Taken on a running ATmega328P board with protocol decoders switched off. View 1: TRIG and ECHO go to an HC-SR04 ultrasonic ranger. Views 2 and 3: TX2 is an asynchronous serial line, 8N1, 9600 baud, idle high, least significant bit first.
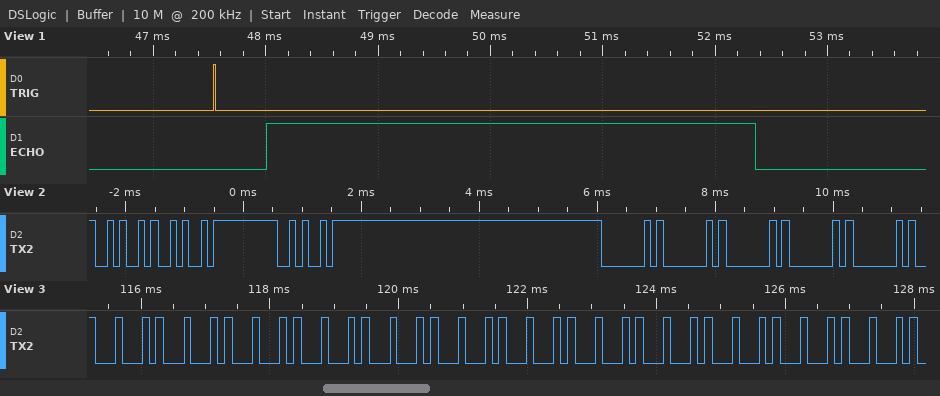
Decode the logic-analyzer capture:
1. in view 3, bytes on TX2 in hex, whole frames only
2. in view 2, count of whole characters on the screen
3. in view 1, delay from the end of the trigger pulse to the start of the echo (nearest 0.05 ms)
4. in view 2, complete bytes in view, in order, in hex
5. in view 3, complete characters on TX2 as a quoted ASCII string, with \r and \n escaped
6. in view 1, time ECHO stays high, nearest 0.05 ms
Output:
44 44 44 44 44 44 44 44 44 44 44 44
8
0.45 ms
4A 4A 4A 40 40 40 40 40
"DDDDDDDDDDDD"
4.35 ms
